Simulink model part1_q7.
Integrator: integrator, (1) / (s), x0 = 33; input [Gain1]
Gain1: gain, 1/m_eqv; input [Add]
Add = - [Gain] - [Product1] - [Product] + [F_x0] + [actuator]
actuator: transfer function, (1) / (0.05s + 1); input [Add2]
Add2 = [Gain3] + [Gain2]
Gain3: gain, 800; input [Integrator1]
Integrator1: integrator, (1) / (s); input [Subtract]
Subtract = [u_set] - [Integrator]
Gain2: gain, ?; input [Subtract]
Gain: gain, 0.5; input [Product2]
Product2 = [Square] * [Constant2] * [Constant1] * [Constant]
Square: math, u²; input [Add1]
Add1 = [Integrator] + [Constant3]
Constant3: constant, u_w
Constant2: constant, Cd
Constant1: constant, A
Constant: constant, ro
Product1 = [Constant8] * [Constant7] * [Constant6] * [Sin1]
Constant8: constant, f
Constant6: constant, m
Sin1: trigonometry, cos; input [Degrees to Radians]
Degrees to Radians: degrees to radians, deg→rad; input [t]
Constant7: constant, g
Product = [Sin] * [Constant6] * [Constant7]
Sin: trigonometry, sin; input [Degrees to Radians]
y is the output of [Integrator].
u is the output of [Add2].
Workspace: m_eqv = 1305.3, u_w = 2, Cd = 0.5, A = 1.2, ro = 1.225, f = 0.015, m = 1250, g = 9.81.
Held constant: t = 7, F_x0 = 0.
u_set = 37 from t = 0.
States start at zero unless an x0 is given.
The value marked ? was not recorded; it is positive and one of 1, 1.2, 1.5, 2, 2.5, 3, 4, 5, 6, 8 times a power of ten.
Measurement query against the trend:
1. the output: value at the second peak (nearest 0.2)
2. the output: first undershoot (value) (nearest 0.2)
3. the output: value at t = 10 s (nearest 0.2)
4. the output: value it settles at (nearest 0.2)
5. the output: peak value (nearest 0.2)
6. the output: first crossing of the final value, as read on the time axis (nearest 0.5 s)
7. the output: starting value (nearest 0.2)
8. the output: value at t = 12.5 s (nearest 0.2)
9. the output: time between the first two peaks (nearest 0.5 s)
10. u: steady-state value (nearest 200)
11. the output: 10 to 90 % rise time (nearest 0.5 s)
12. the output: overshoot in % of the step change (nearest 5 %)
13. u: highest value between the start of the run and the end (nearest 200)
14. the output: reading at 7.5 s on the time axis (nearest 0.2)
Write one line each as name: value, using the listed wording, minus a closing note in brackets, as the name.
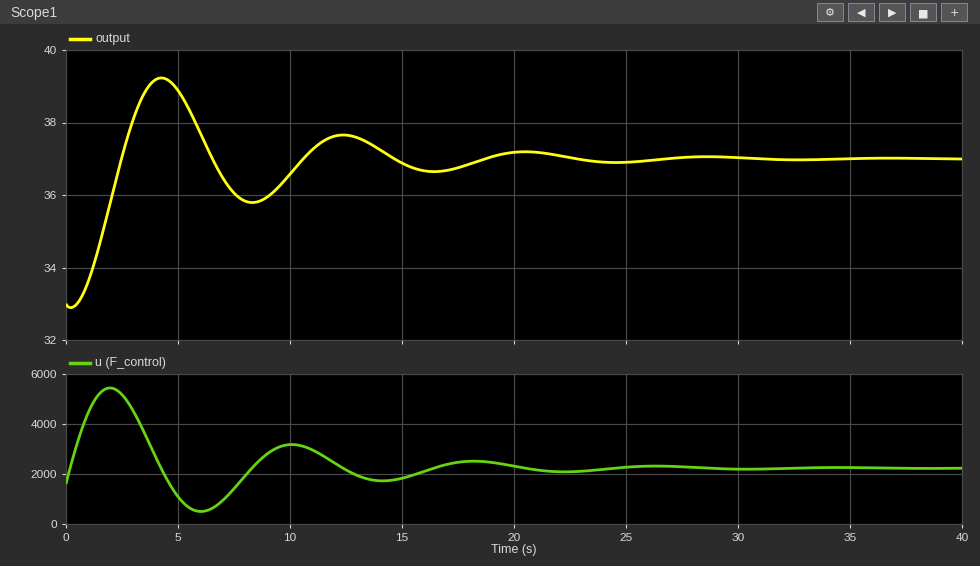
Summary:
the output: value at the second peak: 37.6
the output: first undershoot (value): 35.8
the output: value at t = 10 s: 36.6
the output: value it settles at: 37.0
the output: peak value: 39.2
the output: first crossing of the final value, as read on the time axis: 2.5 s
the output: starting value: 33.0
the output: value at t = 12.5 s: 37.6
the output: time between the first two peaks: 8.0 s
u: steady-state value: 2200
the output: 10 to 90 % rise time: 1.5 s
the output: overshoot in % of the step change: 55 %
u: highest value between the start of the run and the end: 5400
the output: reading at 7.5 s on the time axis: 36.0
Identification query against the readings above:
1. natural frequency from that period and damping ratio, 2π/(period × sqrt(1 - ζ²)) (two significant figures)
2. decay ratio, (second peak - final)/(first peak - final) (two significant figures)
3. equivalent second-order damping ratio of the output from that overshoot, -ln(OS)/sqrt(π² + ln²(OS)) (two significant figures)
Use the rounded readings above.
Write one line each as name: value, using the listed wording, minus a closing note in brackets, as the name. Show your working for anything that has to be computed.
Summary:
natural frequency from that period and damping ratio, 2π/(period × sqrt(1 - ζ²)): 2π / (8 × sqrt(1 - 0.19²)) = 0.80 rad/s
decay ratio, (second peak - final)/(first peak - final): (37.6 - 37) / (39.2 - 37) = 0.27
equivalent second-order damping ratio of the output from that overshoot, -ln(OS)/sqrt(π² + ln²(OS)): ln(0.55) = -0.598; 0.598 / sqrt(9.870 + 0.357) = 0.19
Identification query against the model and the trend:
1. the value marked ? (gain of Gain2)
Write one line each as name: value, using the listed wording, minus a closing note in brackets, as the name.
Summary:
the value marked ?: 400
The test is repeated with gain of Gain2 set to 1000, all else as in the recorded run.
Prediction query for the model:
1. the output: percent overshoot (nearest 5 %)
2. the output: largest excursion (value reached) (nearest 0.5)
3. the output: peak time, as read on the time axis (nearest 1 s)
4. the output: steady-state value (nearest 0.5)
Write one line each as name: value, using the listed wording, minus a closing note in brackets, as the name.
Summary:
the output: percent overshoot: 20 %
the output: largest excursion (value reached): 38.0
the output: peak time, as read on the time axis: 4 s
the output: steady-state value: 37.0
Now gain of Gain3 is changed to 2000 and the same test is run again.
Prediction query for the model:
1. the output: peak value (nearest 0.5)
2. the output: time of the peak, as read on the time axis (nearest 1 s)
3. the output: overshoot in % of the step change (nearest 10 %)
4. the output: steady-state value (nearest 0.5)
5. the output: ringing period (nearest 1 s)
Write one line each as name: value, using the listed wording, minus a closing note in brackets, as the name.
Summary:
the output: peak value: 40.0
the output: time of the peak, as read on the time axis: 3 s
the output: overshoot in % of the step change: 70 %
the output: steady-state value: 37.0
the output: ringing period: 5 s
